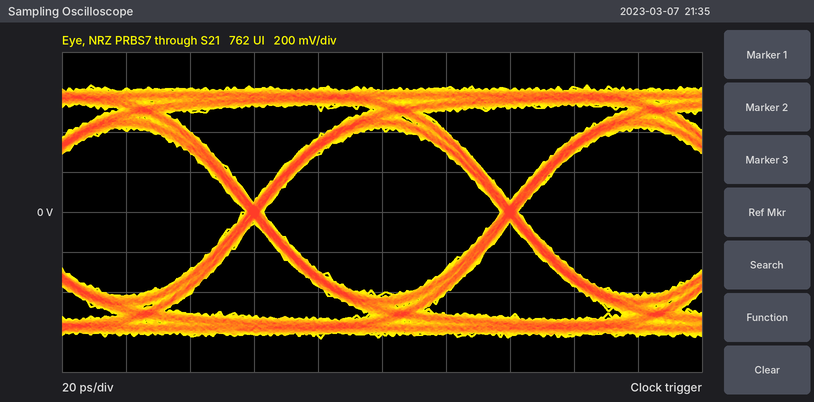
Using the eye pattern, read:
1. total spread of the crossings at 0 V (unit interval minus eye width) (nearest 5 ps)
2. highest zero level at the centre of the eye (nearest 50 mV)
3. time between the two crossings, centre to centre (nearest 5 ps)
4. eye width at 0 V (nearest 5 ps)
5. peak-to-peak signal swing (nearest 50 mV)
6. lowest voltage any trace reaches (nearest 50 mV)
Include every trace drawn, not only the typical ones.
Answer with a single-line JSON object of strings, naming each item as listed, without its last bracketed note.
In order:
{"total spread of the crossings at 0 V (unit interval minus eye width)": "5 ps", "highest zero level at the centre of the eye": "-400 mV", "time between the two crossings, centre to centre": "80 ps", "eye width at 0 V": "75 ps", "peak-to-peak signal swing": "1.25 V", "lowest voltage any trace reaches": "-650 mV"}
